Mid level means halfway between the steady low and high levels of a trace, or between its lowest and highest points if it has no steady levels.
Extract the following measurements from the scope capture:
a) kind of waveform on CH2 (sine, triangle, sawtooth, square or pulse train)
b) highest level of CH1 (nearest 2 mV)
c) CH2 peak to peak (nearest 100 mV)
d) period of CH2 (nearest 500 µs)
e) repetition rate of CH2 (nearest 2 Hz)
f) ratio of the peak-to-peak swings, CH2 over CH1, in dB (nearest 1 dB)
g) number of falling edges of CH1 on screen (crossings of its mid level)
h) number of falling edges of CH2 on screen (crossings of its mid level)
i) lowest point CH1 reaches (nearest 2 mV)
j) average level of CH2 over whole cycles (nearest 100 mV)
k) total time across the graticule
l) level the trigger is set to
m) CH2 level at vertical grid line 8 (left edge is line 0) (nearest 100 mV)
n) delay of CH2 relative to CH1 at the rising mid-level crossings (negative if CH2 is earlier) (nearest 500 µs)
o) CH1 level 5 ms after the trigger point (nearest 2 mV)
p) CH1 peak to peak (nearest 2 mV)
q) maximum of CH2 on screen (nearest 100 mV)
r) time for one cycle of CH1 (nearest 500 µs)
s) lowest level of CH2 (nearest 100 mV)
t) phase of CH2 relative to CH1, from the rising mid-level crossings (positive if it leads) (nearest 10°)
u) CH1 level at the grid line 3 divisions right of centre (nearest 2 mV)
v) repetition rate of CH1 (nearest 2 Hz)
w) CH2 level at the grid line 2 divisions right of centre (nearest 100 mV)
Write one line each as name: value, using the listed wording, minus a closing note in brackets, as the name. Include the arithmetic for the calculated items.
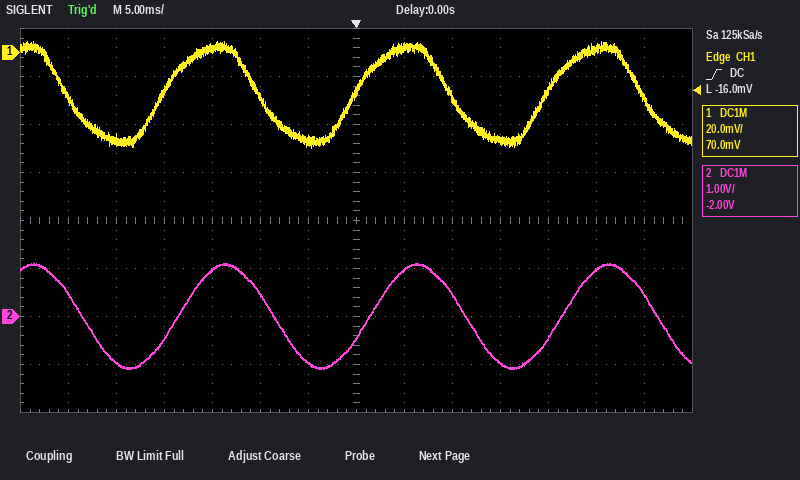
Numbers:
kind of waveform on CH2: sine
highest level of CH1: 4 mV
CH2 peak to peak: 1.1 V − (-1.1 V) = 2.2 V
period of CH2: 20.0 ms
repetition rate of CH2: 1 / 20.0 ms ≈ 50 Hz
ratio of the peak-to-peak swings, CH2 over CH1, in dB: 20 log10(2.2 V / 44 mV) ≈ 34 dB
number of falling edges of CH1 on screen: 4
number of falling edges of CH2 on screen: 4
lowest point CH1 reaches: -40 mV
average level of CH2 over whole cycles: (1.1 V + (-1.1 V)) / 2 ≈ 0.0 V
total time across the graticule: 70 ms
level the trigger is set to: -16.0 mV
CH2 level at vertical grid line 8 (left edge is line 0): 1.0 V
delay of CH2 relative to CH1 at the rising mid-level crossings (negative if CH2 is earlier): +1.5 ms
CH1 level 5 ms after the trigger point: 2 mV
CH1 peak to peak: 4 mV − (-40 mV) = 44 mV
maximum of CH2 on screen: 1.1 V
time for one cycle of CH1: 20.0 ms
lowest level of CH2: -1.1 V
phase of CH2 relative to CH1, from the rising mid-level crossings (positive if it leads): −360° × (+1.5 ms) / 20.0 ms ≈ -27.0°, so -30° to the nearest 10°
CH1 level at the grid line 3 divisions right of centre: -36 mV
repetition rate of CH1: 1 / 20.0 ms ≈ 50 Hz
CH2 level at the grid line 2 divisions right of centre: 500 mV
